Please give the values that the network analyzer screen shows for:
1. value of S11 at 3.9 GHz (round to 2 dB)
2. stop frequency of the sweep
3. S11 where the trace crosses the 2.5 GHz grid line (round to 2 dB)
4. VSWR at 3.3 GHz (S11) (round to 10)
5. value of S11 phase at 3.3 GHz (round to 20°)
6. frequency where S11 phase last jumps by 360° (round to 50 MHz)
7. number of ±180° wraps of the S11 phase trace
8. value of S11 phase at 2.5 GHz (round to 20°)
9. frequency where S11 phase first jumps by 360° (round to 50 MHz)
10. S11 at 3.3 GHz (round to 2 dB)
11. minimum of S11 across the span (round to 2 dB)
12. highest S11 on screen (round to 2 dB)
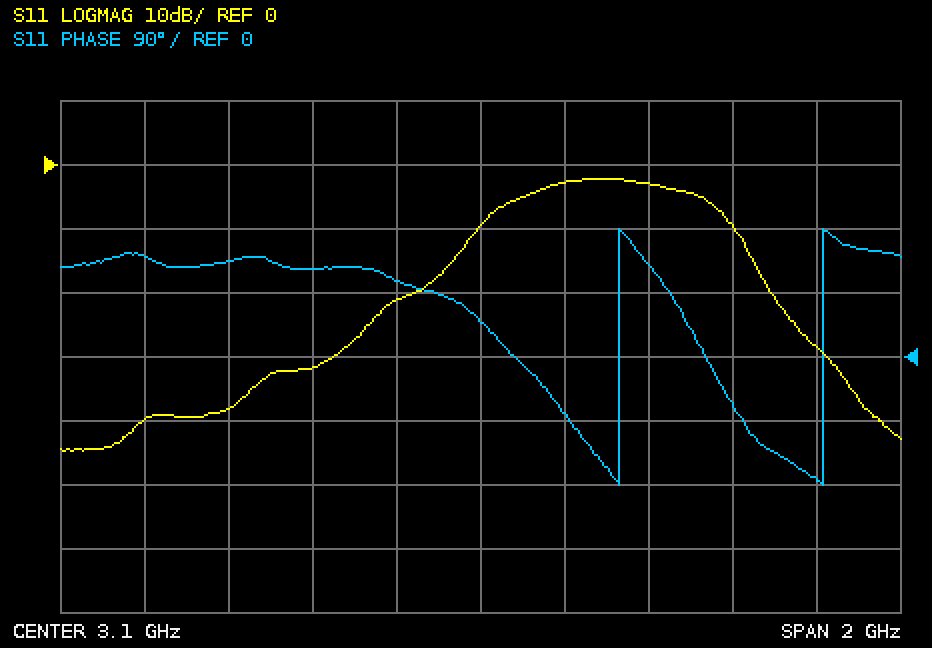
-28 dB
4.1 GHz
-38 dB
10
-80°
3.90 GHz
2
140°
3.45 GHz
-2 dB
-44 dB
-2 dB
